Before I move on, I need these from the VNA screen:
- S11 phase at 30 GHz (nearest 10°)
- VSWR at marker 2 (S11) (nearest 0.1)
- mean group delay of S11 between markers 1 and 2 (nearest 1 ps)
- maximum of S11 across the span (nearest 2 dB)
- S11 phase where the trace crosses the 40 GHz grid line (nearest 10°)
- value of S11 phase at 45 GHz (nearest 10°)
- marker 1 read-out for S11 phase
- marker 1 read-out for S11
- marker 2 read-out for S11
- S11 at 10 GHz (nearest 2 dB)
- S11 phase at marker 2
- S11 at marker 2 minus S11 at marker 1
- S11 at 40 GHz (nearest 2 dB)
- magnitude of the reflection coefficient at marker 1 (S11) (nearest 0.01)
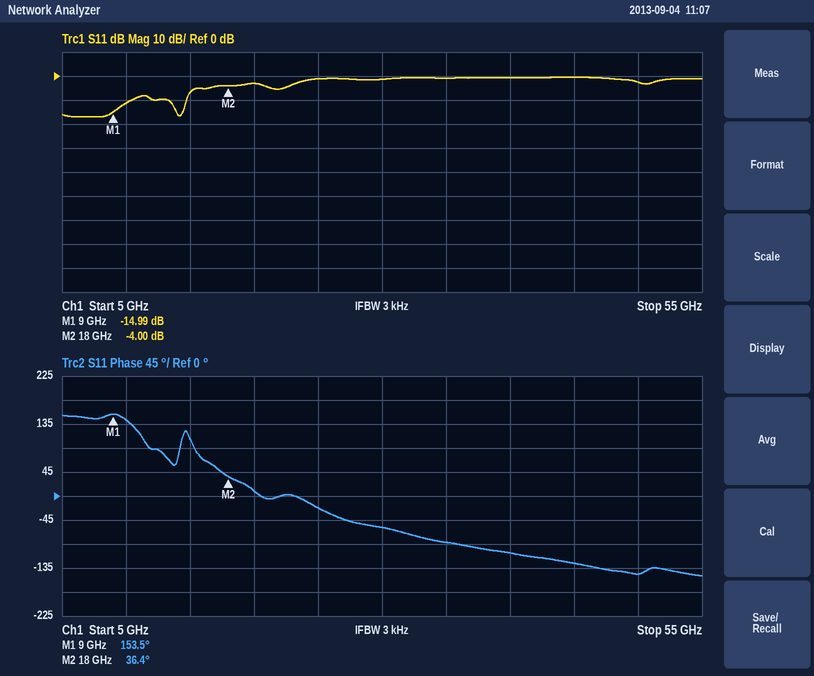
-60°
4.4
36 ps
0 dB
-110°
-130°
153.5°
-14.99 dB
-4.00 dB
-12 dB
36.4°
10.99 dB
0 dB
0.18
